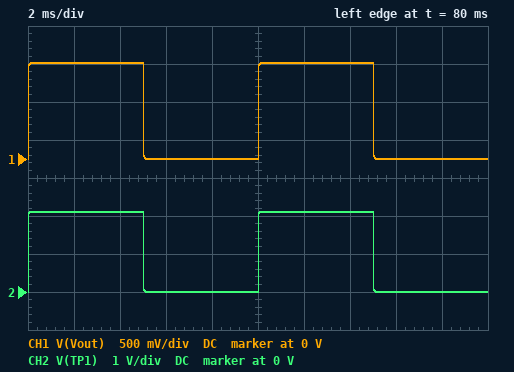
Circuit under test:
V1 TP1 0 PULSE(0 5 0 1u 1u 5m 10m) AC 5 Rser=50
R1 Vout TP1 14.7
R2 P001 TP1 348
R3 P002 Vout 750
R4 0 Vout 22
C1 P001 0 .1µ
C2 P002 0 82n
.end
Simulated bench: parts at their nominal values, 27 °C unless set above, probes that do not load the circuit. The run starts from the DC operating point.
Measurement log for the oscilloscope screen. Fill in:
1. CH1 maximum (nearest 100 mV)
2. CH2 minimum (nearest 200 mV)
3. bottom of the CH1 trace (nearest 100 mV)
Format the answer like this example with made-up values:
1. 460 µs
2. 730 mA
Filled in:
1. 1.3 V
2. 0 V
3. 0 V
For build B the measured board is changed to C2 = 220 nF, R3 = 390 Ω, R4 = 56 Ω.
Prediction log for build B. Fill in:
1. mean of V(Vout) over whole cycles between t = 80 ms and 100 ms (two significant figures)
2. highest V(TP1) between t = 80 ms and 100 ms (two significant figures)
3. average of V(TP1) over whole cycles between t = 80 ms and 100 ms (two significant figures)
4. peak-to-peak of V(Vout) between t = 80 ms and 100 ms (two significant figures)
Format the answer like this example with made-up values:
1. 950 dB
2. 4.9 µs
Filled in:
1. 1.2 V
2. 2.9 V
3. 1.5 V
4. 2.3 V
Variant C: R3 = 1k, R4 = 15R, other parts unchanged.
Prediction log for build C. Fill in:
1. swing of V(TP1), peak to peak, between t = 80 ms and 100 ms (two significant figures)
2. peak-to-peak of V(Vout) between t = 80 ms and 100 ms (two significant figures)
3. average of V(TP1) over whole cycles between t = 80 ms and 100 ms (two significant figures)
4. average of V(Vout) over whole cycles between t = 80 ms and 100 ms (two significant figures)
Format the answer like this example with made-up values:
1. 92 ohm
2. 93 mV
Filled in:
1. 1.9 V
2. 940 mV
3. 930 mV
4. 470 mV
